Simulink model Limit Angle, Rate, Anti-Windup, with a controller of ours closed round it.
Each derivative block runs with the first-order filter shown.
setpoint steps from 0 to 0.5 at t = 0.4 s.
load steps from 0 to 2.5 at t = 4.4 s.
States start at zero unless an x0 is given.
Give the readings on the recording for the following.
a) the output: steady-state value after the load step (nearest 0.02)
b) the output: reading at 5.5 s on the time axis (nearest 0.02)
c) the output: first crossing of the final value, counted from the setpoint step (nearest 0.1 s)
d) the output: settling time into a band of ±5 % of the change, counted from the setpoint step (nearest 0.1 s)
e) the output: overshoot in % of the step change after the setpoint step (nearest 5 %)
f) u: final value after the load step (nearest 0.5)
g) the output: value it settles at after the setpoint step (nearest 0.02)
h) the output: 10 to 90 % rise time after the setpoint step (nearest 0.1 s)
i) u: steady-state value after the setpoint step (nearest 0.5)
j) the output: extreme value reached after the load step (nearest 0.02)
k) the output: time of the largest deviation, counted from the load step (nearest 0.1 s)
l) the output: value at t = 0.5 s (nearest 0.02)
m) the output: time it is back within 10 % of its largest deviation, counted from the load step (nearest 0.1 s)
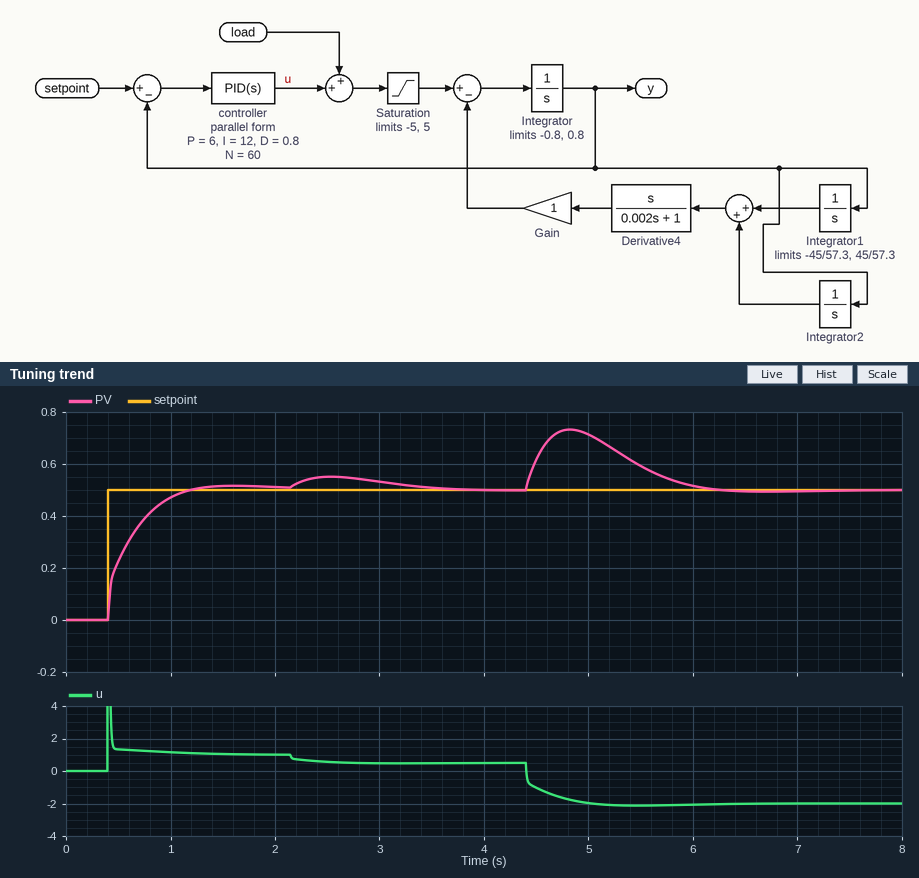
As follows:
0.50
0.60
0.8 s
2.7 s
10 %
-2.0
0.50
0.5 s
0.5
0.74
0.4 s
0.22
1.5 s
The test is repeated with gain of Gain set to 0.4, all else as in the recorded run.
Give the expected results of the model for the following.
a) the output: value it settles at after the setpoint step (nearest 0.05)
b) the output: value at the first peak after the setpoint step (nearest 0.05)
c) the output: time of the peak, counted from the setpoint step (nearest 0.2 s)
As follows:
0.50
0.55
1.0 s
